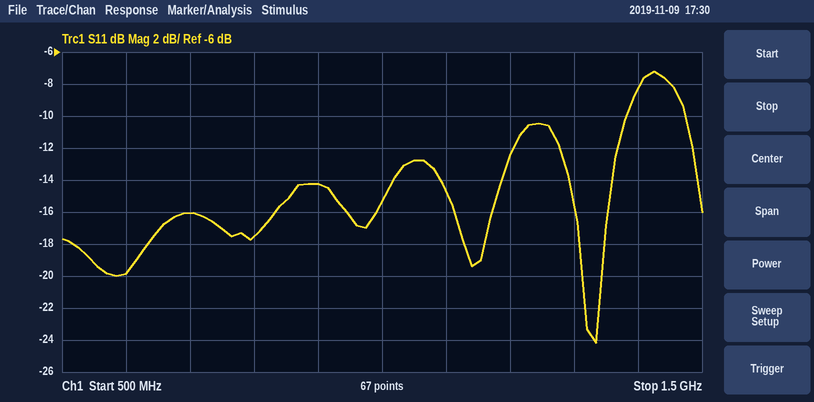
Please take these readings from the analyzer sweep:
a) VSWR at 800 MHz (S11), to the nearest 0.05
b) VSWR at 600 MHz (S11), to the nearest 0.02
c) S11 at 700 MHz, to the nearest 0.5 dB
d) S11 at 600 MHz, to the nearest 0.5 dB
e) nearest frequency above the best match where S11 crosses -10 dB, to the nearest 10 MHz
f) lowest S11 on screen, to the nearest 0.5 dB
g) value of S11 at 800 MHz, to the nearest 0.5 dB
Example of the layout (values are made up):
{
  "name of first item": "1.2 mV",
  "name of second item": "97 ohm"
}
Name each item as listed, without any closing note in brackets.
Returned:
{
  "VSWR at 800 MHz (S11), to the nearest 0.05": "1.30",
  "VSWR at 600 MHz (S11), to the nearest 0.02": "1.22",
  "S11 at 700 MHz, to the nearest 0.5 dB": "-16.0 dB",
  "S11 at 600 MHz, to the nearest 0.5 dB": "-20.0 dB",
  "nearest frequency above the best match where S11 crosses -10 dB, to the nearest 10 MHz": "1.38 GHz",
  "lowest S11 on screen, to the nearest 0.5 dB": "-24.0 dB",
  "value of S11 at 800 MHz, to the nearest 0.5 dB": "-17.5 dB"
}
